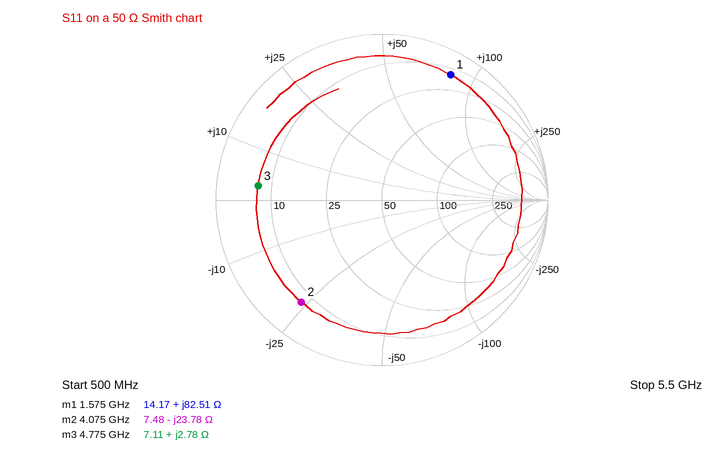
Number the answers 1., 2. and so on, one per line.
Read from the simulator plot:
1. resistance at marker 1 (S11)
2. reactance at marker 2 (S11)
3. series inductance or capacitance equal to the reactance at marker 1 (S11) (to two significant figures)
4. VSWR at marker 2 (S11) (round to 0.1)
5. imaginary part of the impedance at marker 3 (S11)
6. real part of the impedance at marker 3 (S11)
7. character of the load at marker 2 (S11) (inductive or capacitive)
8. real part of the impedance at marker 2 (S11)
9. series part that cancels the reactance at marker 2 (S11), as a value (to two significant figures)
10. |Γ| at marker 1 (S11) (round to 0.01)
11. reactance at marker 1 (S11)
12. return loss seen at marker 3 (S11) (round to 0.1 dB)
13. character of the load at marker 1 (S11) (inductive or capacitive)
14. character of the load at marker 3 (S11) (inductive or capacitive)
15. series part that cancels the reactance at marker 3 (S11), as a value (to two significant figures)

1. 14.17 Ω
2. -23.78 Ω
3. 8.3 nH
4. 8.2
5. +2.78 Ω
6. 7.11 Ω
7. capacitive
8. 7.48 Ω
9. 930 pH
10. 0.86
11. +82.51 Ω
12. 2.5 dB
13. inductive
14. inductive
15. 12 pF
